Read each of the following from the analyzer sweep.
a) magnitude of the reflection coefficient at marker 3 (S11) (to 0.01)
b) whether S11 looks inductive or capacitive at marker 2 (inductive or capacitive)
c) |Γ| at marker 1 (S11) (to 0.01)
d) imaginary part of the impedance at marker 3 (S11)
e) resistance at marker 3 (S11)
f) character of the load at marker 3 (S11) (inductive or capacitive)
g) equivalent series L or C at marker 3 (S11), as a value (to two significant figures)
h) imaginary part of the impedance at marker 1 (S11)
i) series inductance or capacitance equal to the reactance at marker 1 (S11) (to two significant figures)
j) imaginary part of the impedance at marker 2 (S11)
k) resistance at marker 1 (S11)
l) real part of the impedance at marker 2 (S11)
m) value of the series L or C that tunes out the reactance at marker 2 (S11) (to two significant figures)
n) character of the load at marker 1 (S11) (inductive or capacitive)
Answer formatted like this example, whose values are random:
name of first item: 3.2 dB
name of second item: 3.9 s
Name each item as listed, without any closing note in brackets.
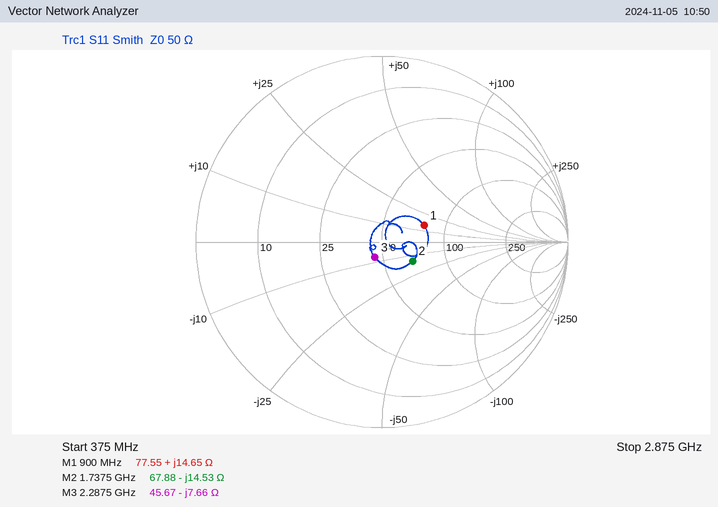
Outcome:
magnitude of the reflection coefficient at marker 3 (S11): 0.09
whether S11 looks inductive or capacitive at marker 2: capacitive
|Γ| at marker 1 (S11): 0.24
imaginary part of the impedance at marker 3: -7.66 Ω
resistance at marker 3: 45.67 Ω
character of the load at marker 3 (S11): capacitive
equivalent series L or C at marker 3 (S11), as a value: 9.1 pF
imaginary part of the impedance at marker 1: +14.65 Ω
series inductance or capacitance equal to the reactance at marker 1 (S11): 2.6 nH
imaginary part of the impedance at marker 2: -14.53 Ω
resistance at marker 1: 77.55 Ω
real part of the impedance at marker 2: 67.88 Ω
value of the series L or C that tunes out the reactance at marker 2 (S11): 1.3 nH
character of the load at marker 1 (S11): inductive
